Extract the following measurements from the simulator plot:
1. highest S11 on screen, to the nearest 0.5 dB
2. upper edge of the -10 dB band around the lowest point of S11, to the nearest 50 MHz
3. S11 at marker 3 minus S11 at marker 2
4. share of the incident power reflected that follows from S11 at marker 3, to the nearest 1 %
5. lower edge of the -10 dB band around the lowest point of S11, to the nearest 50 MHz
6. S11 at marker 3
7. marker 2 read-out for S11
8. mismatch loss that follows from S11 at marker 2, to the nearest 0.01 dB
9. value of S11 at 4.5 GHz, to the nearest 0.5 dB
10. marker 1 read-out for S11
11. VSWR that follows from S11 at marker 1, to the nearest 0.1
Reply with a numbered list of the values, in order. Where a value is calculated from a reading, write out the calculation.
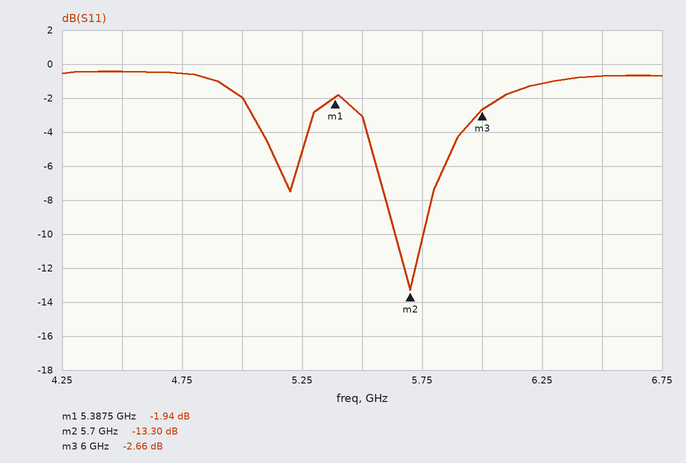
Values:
1. -0.5 dB
2. 5.75 GHz
3. -2.66 − (-13.3) = 10.64 dB
4. 10^(-2.66/10) ≈ 54 %
5. 5.65 GHz
6. -2.66 dB
7. -13.30 dB
8. −10 log10(1 − 10^(-13.3/10)) ≈ 0.21 dB
9. -0.5 dB
10. -1.94 dB
11. (1 + 0.7998)/(1 − 0.7998) ≈ 9.0
